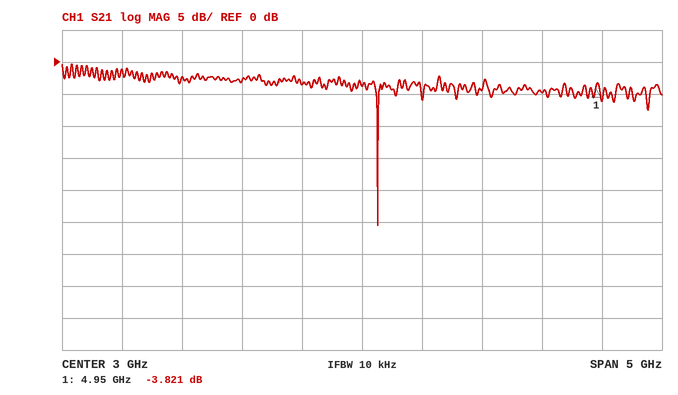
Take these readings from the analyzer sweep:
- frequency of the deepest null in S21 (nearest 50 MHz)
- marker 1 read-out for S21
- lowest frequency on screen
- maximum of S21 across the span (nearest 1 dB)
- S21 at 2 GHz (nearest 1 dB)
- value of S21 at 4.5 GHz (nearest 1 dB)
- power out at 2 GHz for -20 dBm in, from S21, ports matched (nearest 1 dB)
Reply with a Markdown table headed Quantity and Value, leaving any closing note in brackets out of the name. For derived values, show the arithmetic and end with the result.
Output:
| Quantity | Value |
|---|---|
| frequency of the deepest null in S21 | 3.15 GHz |
| marker 1 read-out for S21 | -3.821 dB |
| lowest frequency on screen | 500 MHz |
| maximum of S21 across the span | 0 dB |
| S21 at 2 GHz | -3 dB |
| value of S21 at 4.5 GHz | -5 dB |
| power out at 2 GHz for -20 dBm in, from S21, ports matched | -20 dBm + (-3 dB) = -23 dBm |
